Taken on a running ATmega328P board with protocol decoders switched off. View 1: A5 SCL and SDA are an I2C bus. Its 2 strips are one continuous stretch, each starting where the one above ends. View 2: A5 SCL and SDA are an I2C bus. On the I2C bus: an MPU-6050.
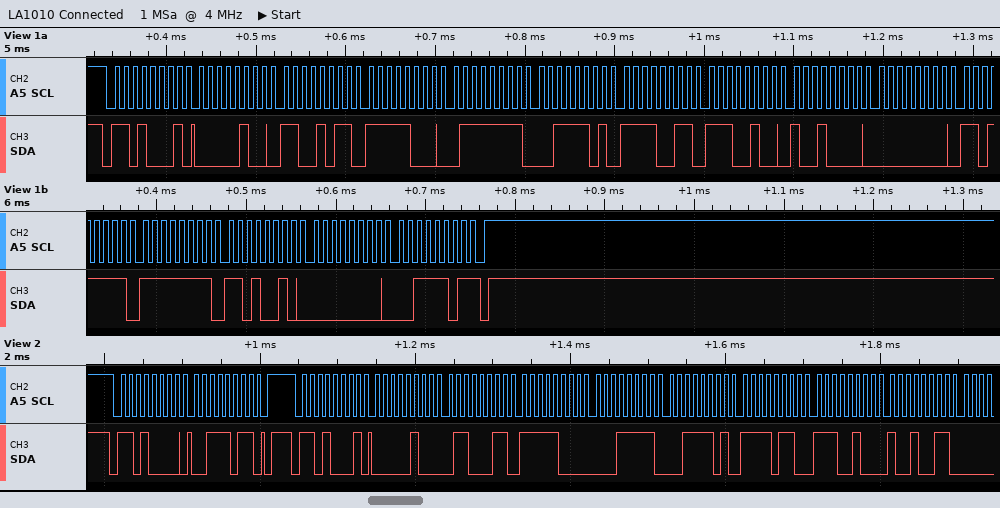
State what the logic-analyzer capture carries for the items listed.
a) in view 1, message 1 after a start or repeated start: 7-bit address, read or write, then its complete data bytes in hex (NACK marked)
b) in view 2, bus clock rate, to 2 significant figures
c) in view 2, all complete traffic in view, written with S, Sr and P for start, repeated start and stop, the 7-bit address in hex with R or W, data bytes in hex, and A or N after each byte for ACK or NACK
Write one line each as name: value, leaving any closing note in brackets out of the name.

in view 1, message 1 after a start or repeated start: 7-bit address, read or write, then its complete data bytes in hex: 0x68 read: 04 CB F8 7F 3D F3 E4 90 00 DF FF D2 00 3D NACK
in view 2, bus clock rate, to 2 significant figures: 100 kHz
in view 2, all complete traffic in view, written with S, Sr and P for start, repeated start and stop, the 7-bit address in hex with R or W, data bytes in hex, and A or N after each byte for ACK or NACK: S 68W A 3B A P S 68R A 04 A 63 A F8 A 1F A 3D A F6 A E4 A 93 A
